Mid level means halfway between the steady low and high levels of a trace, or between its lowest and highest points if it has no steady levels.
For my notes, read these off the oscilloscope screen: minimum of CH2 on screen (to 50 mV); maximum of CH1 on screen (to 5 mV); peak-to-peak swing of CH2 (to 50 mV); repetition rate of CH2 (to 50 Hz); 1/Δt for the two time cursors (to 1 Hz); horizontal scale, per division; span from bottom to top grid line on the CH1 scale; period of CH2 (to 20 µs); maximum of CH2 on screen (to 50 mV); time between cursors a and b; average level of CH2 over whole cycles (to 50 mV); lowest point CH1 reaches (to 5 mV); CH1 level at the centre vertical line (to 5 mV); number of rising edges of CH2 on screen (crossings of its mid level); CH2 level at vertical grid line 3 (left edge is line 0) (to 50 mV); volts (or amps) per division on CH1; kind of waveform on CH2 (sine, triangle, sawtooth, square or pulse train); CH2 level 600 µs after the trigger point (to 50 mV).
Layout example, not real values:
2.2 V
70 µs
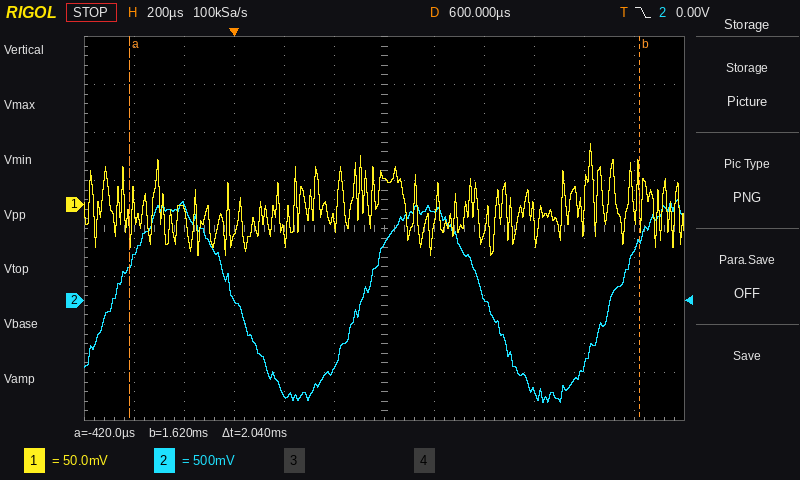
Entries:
-1.05 V
65 mV
2.10 V
1.00 kHz
490 Hz
200 µs
400 mV
1.00 ms
1.05 V
2.04 ms
0 mV
-55 mV
30 mV
3
0 mV
50 mV
sine
600 mV
